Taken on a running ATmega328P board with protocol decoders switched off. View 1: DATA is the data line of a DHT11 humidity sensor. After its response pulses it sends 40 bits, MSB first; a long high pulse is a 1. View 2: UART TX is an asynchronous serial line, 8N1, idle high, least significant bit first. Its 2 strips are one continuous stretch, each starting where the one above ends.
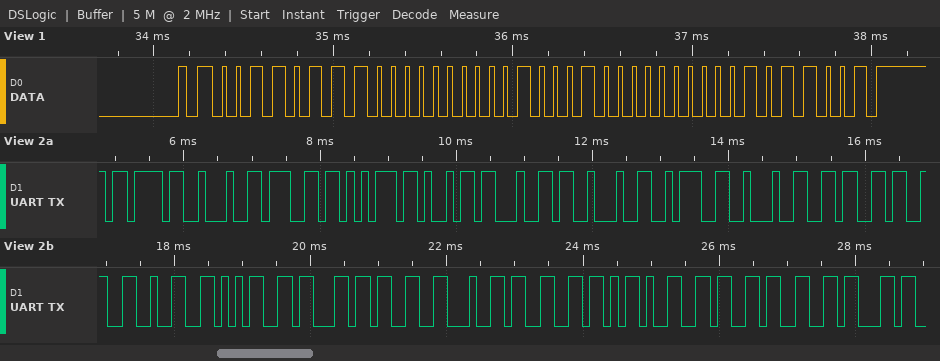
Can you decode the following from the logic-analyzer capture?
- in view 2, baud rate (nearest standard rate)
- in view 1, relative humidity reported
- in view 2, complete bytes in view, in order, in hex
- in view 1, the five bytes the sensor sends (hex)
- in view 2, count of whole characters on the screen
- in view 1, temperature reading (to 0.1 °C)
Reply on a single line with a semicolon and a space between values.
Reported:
9600 baud; 55 %; 7B 22 67 75 69 64 22 3A 22 36 33 32 35 63 33 64 66 2D 36 33 63; 37 00 22 00 59; 21; 34.0 °C
